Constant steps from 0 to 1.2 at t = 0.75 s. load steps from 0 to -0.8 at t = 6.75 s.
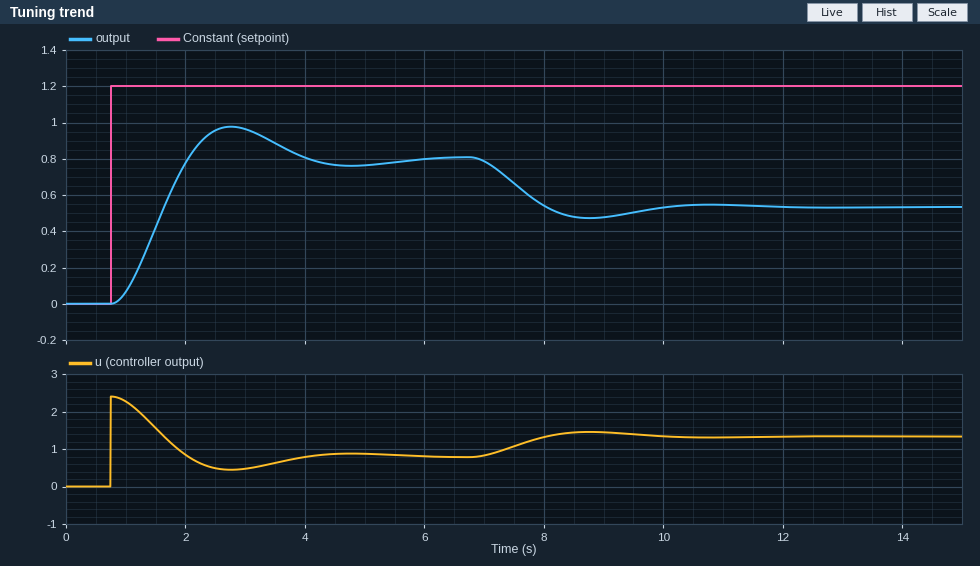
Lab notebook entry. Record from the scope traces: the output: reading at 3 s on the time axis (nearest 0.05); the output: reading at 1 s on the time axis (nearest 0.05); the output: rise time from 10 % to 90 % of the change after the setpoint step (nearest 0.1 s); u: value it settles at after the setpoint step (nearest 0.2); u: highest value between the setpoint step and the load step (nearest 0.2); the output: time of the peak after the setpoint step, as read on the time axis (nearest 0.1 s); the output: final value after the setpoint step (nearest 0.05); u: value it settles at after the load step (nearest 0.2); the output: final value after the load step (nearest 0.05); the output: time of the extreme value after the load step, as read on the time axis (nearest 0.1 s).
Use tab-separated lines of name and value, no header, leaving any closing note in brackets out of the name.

the output: reading at 3 s on the time axis	0.95
the output: reading at 1 s on the time axis	0.05
the output: rise time from 10 % to 90 % of the change after the setpoint step	0.9 s
u: value it settles at after the setpoint step	0.8
u: highest value between the setpoint step and the load step	2.4
the output: time of the peak after the setpoint step, as read on the time axis	2.8 s
the output: final value after the setpoint step	0.80
u: value it settles at after the load step	1.4
the output: final value after the load step	0.55
the output: time of the extreme value after the load step, as read on the time axis	8.8 s
